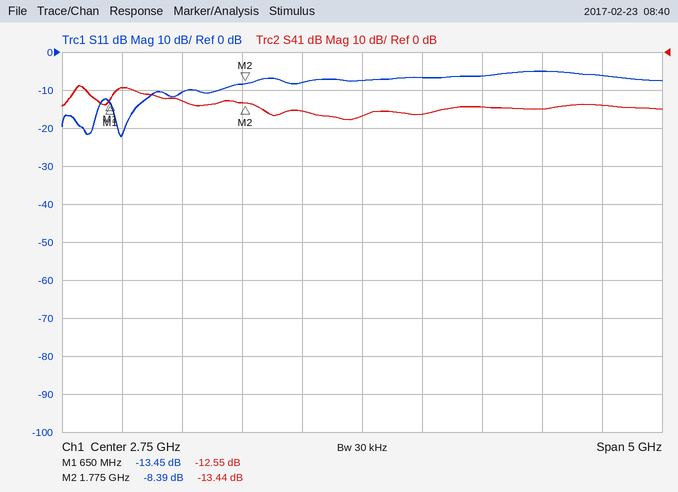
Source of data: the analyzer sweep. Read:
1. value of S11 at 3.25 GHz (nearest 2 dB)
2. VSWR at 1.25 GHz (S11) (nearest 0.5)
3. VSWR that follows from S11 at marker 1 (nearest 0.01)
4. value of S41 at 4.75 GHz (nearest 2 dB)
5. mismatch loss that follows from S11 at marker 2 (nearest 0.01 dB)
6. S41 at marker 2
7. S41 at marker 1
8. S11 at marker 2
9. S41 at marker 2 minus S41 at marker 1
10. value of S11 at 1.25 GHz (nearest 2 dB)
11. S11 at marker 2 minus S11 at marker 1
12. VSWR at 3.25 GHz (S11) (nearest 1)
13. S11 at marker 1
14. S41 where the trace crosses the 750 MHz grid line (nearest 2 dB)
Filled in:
-6 dB
2.0
1.54
-14 dB
0.68 dB
-13.44 dB
-12.55 dB
-8.39 dB
-0.89 dB
-10 dB
5.06 dB
3
-13.45 dB
-10 dB
